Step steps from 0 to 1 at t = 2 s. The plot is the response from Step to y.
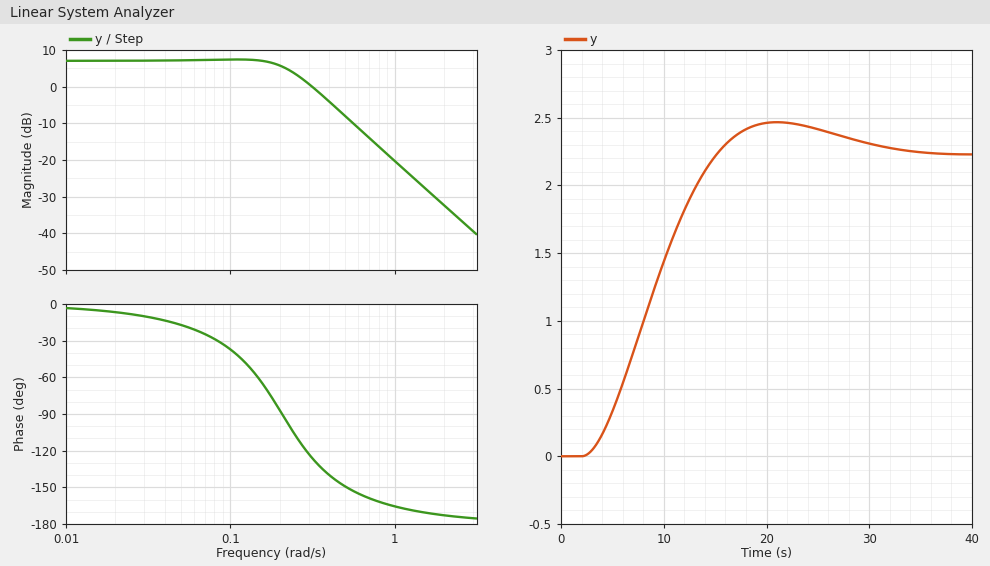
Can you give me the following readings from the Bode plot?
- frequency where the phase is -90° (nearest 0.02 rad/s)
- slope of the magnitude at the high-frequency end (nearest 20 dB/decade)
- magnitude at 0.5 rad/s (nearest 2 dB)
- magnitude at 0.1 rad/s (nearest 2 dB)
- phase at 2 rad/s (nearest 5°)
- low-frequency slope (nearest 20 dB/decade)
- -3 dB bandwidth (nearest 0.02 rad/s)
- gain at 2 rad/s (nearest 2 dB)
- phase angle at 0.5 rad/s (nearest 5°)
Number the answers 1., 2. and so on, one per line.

1. 0.20 rad/s
2. -40 dB/decade
3. -8 dB
4. 8 dB
5. -175°
6. 0 dB/decade
7. 0.24 rad/s
8. -32 dB
9. -150°
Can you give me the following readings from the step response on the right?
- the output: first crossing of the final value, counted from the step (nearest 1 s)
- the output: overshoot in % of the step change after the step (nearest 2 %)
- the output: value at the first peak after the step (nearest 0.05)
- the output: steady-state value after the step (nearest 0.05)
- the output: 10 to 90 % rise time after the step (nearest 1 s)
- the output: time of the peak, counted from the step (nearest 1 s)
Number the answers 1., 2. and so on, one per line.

1. 13 s
2. 10 %
3. 2.45
4. 2.25
5. 9 s
6. 19 s
